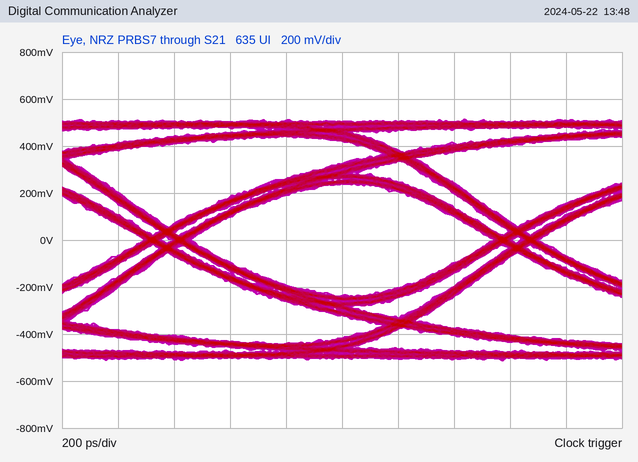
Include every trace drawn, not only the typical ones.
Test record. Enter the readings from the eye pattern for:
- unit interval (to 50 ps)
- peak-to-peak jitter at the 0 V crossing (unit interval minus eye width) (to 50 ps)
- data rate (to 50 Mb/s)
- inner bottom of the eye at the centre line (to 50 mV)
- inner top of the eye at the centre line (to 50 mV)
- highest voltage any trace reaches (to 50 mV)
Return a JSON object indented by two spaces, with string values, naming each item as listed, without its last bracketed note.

{
  "unit interval": "1.25 ns",
  "peak-to-peak jitter at the 0 V crossing (unit interval minus eye width)": "150 ps",
  "data rate": "800 Mb/s",
  "inner bottom of the eye at the centre line": "-250 mV",
  "inner top of the eye at the centre line": "250 mV",
  "highest voltage any trace reaches": "500 mV"
}
